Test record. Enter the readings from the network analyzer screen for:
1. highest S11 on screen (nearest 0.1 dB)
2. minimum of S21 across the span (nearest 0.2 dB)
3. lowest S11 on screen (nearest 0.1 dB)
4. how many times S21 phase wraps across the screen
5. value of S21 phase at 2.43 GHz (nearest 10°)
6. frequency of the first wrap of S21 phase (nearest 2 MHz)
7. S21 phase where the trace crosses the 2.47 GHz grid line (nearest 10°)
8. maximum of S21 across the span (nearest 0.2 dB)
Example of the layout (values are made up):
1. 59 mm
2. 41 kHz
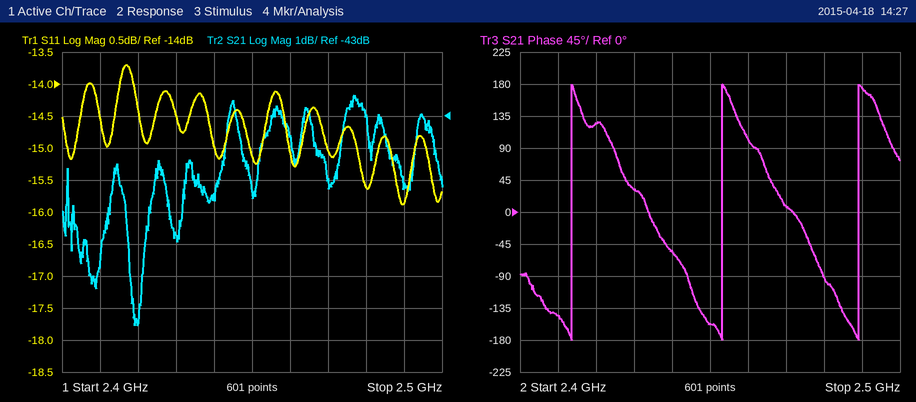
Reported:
1. -13.7 dB
2. -49.6 dB
3. -15.9 dB
4. 3
5. 30°
6. 2.414 GHz
7. 10°
8. -42.4 dB
